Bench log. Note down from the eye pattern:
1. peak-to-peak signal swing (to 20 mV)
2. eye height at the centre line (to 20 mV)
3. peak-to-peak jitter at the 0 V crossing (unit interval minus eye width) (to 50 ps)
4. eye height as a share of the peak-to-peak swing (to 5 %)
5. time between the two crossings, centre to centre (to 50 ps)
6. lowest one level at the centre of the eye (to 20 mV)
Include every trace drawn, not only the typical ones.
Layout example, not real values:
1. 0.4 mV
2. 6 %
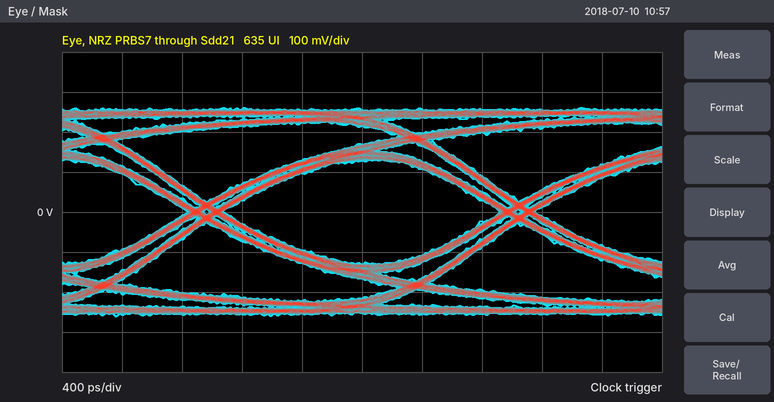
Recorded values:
1. 520 mV
2. 260 mV
3. 250 ps
4. 50 %
5. 2.10 ns
6. 120 mV
